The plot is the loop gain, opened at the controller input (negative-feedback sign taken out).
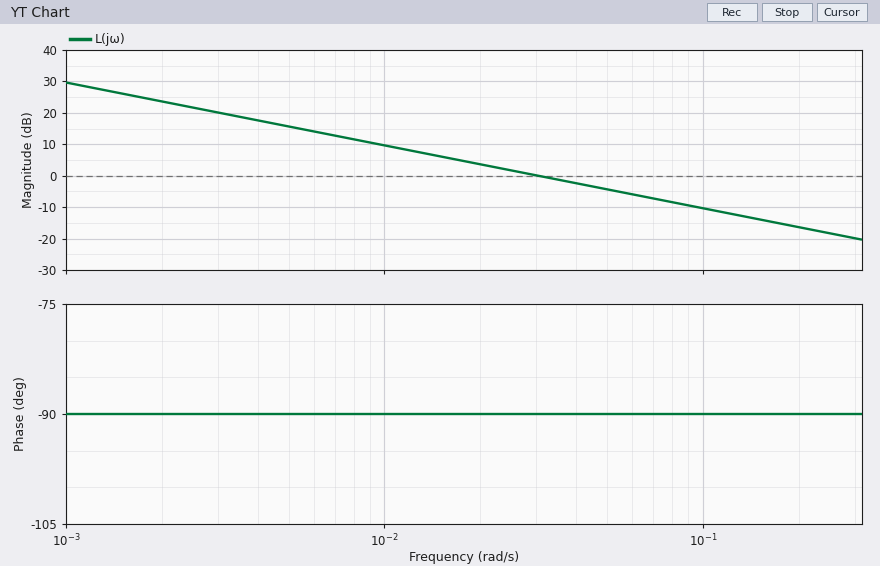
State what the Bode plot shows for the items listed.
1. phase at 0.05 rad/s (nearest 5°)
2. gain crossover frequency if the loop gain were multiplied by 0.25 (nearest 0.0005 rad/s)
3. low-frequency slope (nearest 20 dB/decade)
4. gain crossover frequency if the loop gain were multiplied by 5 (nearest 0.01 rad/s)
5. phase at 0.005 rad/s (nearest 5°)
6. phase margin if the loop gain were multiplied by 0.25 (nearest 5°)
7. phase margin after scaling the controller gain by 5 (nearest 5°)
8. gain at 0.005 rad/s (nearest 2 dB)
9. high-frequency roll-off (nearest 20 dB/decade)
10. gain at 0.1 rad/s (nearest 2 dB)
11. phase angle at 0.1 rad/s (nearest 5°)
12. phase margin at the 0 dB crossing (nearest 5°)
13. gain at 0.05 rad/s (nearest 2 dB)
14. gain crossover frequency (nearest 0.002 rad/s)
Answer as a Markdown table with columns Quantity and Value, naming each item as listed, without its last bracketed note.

| Quantity | Value |
|---|---|
| phase at 0.05 rad/s | -90° |
| gain crossover frequency if the loop gain were multiplied by 0.25 | 0.0075 rad/s |
| low-frequency slope | -20 dB/decade |
| gain crossover frequency if the loop gain were multiplied by 5 | 0.15 rad/s |
| phase at 0.005 rad/s | -90° |
| phase margin if the loop gain were multiplied by 0.25 | 90° |
| phase margin after scaling the controller gain by 5 | 90° |
| gain at 0.005 rad/s | 16 dB |
| high-frequency roll-off | -20 dB/decade |
| gain at 0.1 rad/s | -10 dB |
| phase angle at 0.1 rad/s | -90° |
| phase margin at the 0 dB crossing | 90° |
| gain at 0.05 rad/s | -4 dB |
| gain crossover frequency | 0.030 rad/s |
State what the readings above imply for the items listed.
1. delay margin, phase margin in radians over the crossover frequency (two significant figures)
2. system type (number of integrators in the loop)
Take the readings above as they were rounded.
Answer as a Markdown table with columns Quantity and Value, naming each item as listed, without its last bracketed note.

| Quantity | Value |
|---|---|
| delay margin, phase margin in radians over the crossover frequency | 52 s |
| system type | 1 |
